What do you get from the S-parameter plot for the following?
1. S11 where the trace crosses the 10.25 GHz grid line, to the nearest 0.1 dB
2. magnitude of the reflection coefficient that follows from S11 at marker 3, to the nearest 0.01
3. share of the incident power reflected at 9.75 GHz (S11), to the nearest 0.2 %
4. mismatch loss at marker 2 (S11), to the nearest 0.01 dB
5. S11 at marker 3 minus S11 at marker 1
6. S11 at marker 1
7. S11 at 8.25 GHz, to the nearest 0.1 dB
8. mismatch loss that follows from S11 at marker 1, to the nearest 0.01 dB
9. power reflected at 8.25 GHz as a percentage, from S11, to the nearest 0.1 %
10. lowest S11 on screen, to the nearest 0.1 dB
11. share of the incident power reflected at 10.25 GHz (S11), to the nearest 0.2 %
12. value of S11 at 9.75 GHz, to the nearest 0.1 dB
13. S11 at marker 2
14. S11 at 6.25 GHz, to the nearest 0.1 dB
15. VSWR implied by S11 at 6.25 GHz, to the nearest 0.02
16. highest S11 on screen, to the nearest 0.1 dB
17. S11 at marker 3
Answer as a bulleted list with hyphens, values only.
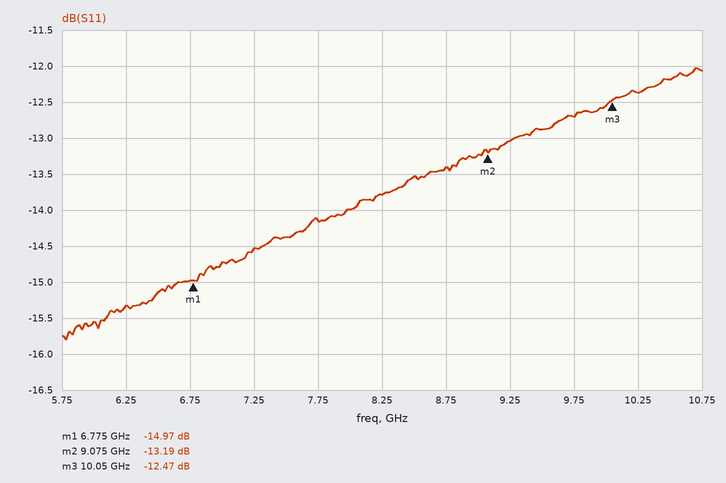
- -12.4 dB
- 0.24
- 5.4 %
- 0.21 dB
- 2.50 dB
- -14.97 dB
- -13.8 dB
- 0.14 dB
- 4.2 %
- -15.8 dB
- 5.8 %
- -12.7 dB
- -13.19 dB
- -15.3 dB
- 1.42
- -12.0 dB
- -12.47 dB
